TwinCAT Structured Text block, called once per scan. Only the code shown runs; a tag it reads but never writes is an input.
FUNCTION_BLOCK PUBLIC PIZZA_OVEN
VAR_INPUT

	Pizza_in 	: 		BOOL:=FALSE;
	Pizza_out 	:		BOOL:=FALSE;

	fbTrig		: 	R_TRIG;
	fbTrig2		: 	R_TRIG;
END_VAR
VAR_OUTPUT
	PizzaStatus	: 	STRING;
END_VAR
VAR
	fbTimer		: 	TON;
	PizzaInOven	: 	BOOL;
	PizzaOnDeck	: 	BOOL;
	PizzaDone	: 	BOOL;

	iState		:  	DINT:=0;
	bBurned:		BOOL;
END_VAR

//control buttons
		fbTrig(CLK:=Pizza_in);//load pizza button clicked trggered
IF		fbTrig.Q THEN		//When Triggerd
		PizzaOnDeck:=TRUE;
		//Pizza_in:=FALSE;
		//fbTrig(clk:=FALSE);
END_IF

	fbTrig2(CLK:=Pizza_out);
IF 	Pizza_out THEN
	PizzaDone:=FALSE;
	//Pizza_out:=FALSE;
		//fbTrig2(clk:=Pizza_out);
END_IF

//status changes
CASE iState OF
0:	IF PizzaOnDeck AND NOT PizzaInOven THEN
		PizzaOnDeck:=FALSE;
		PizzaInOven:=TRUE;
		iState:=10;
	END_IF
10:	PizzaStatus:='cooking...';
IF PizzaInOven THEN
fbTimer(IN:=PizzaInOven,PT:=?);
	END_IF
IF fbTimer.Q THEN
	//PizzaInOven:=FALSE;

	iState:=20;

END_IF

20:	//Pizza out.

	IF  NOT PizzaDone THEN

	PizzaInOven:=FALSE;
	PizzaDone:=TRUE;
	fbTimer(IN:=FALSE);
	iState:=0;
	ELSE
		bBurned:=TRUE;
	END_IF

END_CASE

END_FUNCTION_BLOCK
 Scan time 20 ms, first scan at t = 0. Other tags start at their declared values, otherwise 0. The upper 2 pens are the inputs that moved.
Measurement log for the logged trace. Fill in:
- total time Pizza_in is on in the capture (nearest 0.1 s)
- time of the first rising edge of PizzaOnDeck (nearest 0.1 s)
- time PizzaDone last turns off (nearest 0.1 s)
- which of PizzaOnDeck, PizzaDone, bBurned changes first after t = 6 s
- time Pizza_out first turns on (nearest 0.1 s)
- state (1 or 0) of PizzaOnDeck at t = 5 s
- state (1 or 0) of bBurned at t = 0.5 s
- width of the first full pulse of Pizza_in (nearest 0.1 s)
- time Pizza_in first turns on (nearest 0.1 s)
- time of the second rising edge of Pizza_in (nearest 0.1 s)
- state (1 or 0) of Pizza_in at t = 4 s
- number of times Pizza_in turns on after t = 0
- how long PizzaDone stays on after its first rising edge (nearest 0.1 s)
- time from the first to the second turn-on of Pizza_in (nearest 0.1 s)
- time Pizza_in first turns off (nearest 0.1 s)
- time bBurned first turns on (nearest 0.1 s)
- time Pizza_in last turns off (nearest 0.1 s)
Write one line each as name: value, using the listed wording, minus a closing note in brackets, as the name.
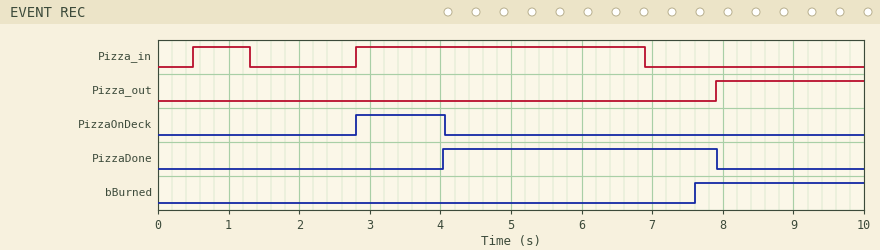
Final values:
total time Pizza_in is on in the capture: 4.9 s
time of the first rising edge of PizzaOnDeck: 2.8 s
time PizzaDone last turns off: 7.9 s
which of PizzaOnDeck, PizzaDone, bBurned changes first after t = 6 s: bBurned
time Pizza_out first turns on: 7.9 s
state (1 or 0) of PizzaOnDeck at t = 5 s: 0
state (1 or 0) of bBurned at t = 0.5 s: 0
width of the first full pulse of Pizza_in: 0.8 s
time Pizza_in first turns on: 0.5 s
time of the second rising edge of Pizza_in: 2.8 s
state (1 or 0) of Pizza_in at t = 4 s: 1
number of times Pizza_in turns on after t = 0: 2
how long PizzaDone stays on after its first rising edge: 3.9 s
time from the first to the second turn-on of Pizza_in: 2.3 s
time Pizza_in first turns off: 1.3 s
time bBurned first turns on: 7.6 s
time Pizza_in last turns off: 6.9 s
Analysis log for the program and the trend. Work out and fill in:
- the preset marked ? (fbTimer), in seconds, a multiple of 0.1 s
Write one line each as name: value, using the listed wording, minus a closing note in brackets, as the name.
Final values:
the preset marked ? (fbTimer), in seconds, a multiple of 0.1 s: 3.5 s
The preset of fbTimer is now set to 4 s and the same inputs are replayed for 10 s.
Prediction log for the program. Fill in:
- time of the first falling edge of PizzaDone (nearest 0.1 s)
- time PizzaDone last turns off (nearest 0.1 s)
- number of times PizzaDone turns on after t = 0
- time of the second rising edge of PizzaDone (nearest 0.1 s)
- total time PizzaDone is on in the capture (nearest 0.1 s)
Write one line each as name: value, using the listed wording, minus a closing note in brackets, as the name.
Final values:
time of the first falling edge of PizzaDone: 7.9 s
time PizzaDone last turns off: 8.6 s
number of times PizzaDone turns on after t = 0: 2
time of the second rising edge of PizzaDone: 8.6 s
total time PizzaDone is on in the capture: 3.4 s
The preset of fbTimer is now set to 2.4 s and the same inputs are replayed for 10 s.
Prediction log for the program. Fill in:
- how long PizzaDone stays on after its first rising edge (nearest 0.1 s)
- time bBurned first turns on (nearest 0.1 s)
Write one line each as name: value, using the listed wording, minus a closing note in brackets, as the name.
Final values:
how long PizzaDone stays on after its first rising edge: 5.0 s
time bBurned first turns on: 5.4 s
